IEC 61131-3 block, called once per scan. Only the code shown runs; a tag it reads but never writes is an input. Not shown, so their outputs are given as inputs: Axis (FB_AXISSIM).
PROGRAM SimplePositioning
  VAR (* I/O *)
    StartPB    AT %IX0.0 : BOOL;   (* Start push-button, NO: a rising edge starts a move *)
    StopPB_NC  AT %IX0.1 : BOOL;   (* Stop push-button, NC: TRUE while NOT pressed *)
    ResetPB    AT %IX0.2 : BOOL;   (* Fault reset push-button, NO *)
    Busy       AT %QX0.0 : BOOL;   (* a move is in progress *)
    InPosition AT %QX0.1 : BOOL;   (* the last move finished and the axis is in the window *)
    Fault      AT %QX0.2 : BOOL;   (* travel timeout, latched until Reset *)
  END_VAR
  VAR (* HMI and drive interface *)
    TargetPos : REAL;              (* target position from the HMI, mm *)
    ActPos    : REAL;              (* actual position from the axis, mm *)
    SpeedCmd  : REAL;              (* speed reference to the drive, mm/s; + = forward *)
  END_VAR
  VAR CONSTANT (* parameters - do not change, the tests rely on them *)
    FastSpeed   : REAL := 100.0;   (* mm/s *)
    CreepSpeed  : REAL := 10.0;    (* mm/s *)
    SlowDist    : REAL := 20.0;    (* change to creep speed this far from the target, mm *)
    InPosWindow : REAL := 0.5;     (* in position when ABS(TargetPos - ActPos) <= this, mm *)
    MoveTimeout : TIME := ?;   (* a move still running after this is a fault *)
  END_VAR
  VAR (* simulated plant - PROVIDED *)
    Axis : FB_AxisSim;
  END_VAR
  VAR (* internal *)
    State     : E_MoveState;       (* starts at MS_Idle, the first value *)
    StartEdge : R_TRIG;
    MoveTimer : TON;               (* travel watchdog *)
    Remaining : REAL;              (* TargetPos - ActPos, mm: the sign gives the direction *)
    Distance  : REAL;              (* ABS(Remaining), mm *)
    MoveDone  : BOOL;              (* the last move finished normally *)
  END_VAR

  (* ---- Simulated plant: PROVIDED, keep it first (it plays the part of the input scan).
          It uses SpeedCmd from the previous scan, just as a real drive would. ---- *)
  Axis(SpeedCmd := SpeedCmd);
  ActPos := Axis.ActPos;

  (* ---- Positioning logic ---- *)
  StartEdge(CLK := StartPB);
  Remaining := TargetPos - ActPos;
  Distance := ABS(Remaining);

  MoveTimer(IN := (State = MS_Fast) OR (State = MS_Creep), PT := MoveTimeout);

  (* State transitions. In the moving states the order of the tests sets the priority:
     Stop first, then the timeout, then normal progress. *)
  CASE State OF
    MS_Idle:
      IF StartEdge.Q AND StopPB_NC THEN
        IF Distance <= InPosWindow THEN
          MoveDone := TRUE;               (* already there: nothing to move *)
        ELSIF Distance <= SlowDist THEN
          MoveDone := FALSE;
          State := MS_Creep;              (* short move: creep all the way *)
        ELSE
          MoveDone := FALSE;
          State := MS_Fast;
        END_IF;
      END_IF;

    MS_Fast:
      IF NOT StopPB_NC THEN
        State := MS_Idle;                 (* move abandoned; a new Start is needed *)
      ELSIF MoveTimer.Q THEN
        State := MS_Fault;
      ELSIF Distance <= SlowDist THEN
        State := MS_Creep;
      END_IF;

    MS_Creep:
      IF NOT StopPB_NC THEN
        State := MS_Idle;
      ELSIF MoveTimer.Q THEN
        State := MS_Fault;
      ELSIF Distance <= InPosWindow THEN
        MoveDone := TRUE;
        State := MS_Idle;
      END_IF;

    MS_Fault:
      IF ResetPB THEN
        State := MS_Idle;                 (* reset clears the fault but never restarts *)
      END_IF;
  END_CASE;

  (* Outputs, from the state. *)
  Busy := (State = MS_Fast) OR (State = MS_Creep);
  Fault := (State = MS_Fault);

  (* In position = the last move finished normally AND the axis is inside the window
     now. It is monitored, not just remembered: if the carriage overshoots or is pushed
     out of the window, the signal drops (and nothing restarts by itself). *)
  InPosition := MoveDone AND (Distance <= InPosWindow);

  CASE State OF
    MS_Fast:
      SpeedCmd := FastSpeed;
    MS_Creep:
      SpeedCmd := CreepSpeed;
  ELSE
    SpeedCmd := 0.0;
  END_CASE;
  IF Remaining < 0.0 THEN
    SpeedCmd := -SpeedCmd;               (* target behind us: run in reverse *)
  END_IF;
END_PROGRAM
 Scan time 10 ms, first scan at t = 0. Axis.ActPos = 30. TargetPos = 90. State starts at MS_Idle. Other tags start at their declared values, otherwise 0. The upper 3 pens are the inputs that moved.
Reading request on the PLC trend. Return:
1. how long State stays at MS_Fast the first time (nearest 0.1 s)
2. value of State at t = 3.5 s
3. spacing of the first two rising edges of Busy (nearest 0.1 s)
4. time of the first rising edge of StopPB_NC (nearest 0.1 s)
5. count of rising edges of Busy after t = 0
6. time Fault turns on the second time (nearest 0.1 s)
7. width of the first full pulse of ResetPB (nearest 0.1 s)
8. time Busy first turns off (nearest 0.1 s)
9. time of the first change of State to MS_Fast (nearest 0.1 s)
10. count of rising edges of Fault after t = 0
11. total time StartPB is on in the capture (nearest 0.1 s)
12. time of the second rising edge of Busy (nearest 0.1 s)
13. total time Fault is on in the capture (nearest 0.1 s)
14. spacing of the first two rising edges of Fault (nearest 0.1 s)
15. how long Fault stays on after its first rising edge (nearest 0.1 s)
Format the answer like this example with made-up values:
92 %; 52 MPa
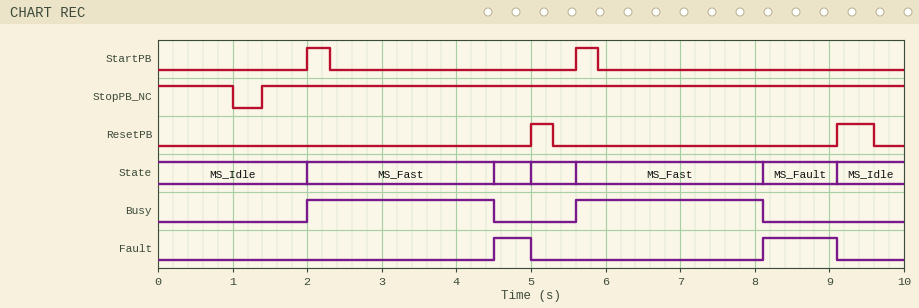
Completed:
2.5 s; MS_Fast; 3.6 s; 1.4 s; 2; 8.1 s; 0.3 s; 4.5 s; 2.0 s; 2; 0.6 s; 5.6 s; 1.5 s; 3.6 s; 0.5 s
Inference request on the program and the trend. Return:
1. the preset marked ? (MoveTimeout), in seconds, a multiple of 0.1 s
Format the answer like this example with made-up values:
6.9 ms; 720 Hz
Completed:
2.5 s
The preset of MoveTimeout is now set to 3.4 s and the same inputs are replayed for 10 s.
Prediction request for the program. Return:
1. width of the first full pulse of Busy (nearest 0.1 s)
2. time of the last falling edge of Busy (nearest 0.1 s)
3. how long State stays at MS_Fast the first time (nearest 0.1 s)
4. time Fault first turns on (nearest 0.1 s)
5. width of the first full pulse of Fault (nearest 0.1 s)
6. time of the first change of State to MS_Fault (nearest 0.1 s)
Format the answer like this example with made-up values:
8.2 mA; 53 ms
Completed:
3.4 s; 5.4 s; 3.4 s; 5.4 s; 3.7 s; 5.4 s
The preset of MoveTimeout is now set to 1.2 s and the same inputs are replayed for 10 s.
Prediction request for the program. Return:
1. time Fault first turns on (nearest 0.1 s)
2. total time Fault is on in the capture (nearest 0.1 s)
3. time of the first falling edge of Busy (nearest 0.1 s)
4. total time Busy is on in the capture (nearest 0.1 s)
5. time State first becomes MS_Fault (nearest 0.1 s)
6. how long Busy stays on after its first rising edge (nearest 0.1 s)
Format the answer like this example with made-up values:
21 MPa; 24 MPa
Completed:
3.2 s; 4.1 s; 3.2 s; 2.4 s; 3.2 s; 1.2 s
